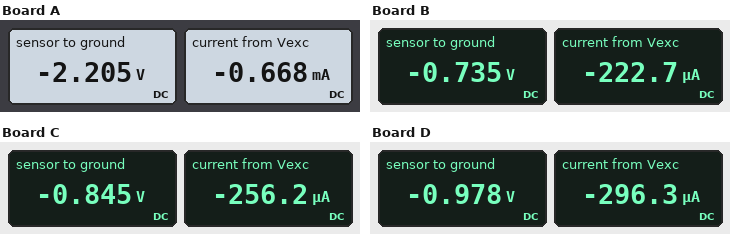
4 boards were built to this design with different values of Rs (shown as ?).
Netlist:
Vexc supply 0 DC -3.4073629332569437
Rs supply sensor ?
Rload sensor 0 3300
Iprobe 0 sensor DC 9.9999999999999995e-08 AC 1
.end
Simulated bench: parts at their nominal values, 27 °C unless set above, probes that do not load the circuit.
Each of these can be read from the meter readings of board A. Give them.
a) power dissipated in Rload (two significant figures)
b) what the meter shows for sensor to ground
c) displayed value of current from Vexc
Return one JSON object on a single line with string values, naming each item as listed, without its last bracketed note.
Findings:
{"power dissipated in Rload": "1.5 mW", "what the meter shows for sensor to ground": "-2.205 V", "displayed value of current from Vexc": "-0.668 mA"}
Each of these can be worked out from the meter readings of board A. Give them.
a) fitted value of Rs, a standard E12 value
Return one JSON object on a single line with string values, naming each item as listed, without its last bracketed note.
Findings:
{"fitted value of Rs, a standard E12 value": "1.8 kΩ"}
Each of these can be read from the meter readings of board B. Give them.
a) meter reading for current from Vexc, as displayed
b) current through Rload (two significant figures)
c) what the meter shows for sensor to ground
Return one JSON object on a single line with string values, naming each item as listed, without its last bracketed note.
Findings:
{"meter reading for current from Vexc, as displayed": "-222.7 µA", "current through Rload": "220 µA", "what the meter shows for sensor to ground": "-0.735 V"}
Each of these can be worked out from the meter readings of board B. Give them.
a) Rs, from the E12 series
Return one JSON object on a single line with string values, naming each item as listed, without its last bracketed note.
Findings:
{"Rs, from the E12 series": "12 kΩ"}
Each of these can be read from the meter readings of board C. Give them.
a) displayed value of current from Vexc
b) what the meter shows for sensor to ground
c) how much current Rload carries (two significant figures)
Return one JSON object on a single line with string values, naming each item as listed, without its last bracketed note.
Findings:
{"displayed value of current from Vexc": "-256.2 µA", "what the meter shows for sensor to ground": "-0.845 V", "how much current Rload carries": "260 µA"}
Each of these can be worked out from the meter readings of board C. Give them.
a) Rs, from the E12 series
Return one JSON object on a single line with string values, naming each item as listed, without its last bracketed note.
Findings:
{"Rs, from the E12 series": "10 kΩ"}
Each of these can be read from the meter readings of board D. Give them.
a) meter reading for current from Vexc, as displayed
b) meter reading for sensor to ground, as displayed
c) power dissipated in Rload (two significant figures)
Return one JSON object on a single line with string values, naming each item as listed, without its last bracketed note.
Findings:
{"meter reading for current from Vexc, as displayed": "-296.3 µA", "meter reading for sensor to ground, as displayed": "-0.978 V", "power dissipated in Rload": "290 µW"}
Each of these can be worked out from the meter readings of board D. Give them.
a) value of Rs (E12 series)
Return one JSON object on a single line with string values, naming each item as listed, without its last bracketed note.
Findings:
{"value of Rs": "8.2 kΩ"}
